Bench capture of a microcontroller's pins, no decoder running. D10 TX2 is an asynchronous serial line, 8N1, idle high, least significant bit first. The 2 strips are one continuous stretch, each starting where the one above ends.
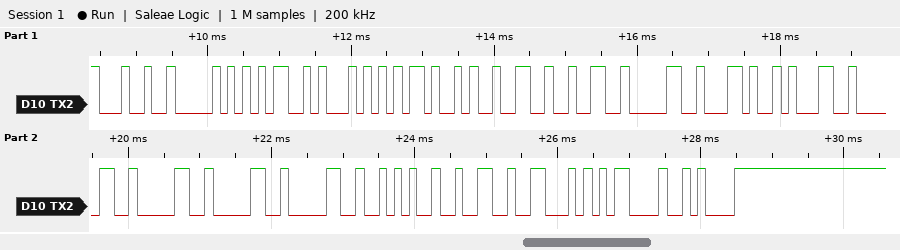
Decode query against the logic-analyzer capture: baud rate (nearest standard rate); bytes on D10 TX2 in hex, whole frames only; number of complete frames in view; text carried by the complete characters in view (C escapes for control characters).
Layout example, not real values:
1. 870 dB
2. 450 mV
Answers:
1. 9600 baud
2. 24 50 4D 54 4B 32 32 30 2C 31 30 30 30 30 2A 32 46 0D 0A
3. 19
4. "$PMTK220,10000*2F\r\n"
